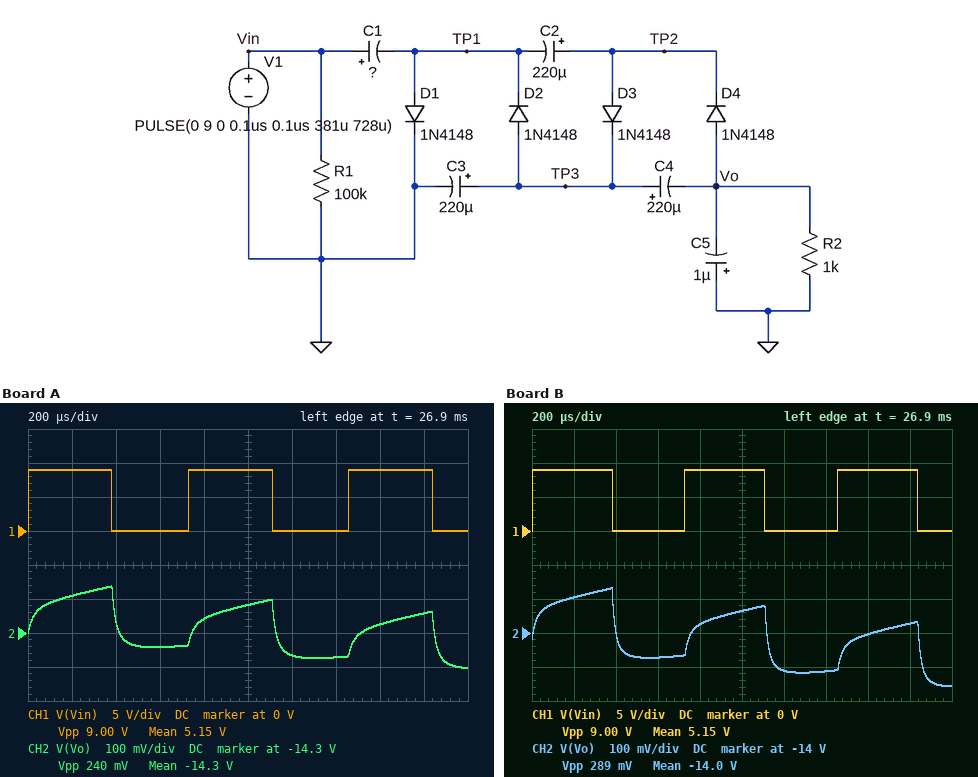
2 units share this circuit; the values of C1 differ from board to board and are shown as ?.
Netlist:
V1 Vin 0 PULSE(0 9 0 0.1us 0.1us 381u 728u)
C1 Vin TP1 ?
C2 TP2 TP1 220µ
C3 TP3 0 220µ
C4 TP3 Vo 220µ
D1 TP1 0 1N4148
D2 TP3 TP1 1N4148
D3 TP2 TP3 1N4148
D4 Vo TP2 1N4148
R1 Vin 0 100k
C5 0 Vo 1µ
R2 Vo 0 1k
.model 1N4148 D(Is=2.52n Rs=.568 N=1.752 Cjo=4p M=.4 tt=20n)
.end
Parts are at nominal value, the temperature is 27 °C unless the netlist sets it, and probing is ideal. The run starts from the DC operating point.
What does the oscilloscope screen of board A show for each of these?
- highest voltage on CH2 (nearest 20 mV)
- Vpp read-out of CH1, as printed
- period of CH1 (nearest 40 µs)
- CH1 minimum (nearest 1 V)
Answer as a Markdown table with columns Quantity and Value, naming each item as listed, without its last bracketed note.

| Quantity | Value |
|---|---|
| highest voltage on CH2 | -14.16 V |
| Vpp read-out of CH1, as printed | 9.00 V |
| period of CH1 | 720 µs |
| CH1 minimum | 0 V |
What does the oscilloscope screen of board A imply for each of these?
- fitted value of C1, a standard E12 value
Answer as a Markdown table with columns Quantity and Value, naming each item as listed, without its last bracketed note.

| Quantity | Value |
|---|---|
| fitted value of C1, a standard E12 value | 82 µF |
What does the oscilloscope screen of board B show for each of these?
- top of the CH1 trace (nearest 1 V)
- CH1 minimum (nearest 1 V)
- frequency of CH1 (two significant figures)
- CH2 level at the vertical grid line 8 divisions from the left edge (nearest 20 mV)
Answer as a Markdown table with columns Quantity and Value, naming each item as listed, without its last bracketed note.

| Quantity | Value |
|---|---|
| top of the CH1 trace | 9 V |
| CH1 minimum | 0 V |
| frequency of CH1 | 1.4 kHz |
| CH2 level at the vertical grid line 8 divisions from the left edge | -14.00 V |
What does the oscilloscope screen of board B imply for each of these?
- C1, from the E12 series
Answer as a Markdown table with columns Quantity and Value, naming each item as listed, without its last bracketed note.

| Quantity | Value |
|---|---|
| C1, from the E12 series | 68 µF |
